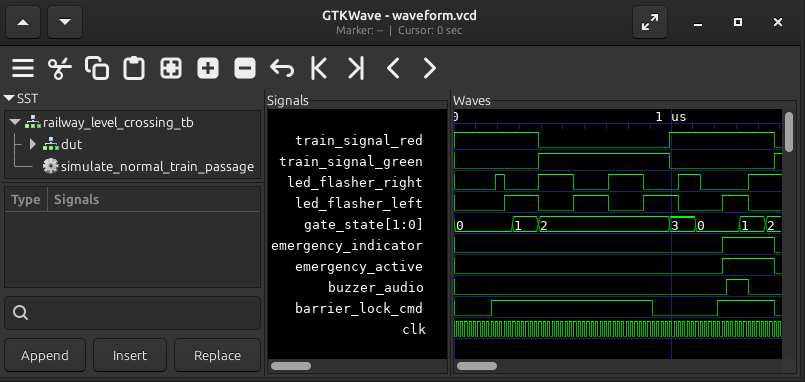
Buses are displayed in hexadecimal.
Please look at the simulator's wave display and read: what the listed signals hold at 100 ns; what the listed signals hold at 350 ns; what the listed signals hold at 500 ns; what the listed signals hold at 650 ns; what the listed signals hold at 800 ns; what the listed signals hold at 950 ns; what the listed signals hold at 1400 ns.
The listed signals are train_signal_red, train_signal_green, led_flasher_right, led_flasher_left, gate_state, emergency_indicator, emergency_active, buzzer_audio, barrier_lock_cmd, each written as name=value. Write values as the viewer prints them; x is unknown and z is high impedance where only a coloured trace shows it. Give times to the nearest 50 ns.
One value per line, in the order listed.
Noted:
train_signal_red=1, train_signal_green=0, led_flasher_right=0, led_flasher_left=0, gate_state=0, emergency_indicator=0, emergency_active=0, buzzer_audio=0, barrier_lock_cmd=0
train_signal_red=1, train_signal_green=0, led_flasher_right=0, led_flasher_left=1, gate_state=1, emergency_indicator=0, emergency_active=0, buzzer_audio=0, barrier_lock_cmd=1
train_signal_red=0, train_signal_green=1, led_flasher_right=1, led_flasher_left=0, gate_state=2, emergency_indicator=0, emergency_active=0, buzzer_audio=0, barrier_lock_cmd=1
train_signal_red=0, train_signal_green=1, led_flasher_right=0, led_flasher_left=1, gate_state=2, emergency_indicator=0, emergency_active=0, buzzer_audio=0, barrier_lock_cmd=1
train_signal_red=0, train_signal_green=1, led_flasher_right=1, led_flasher_left=0, gate_state=2, emergency_indicator=0, emergency_active=0, buzzer_audio=0, barrier_lock_cmd=1
train_signal_red=0, train_signal_green=1, led_flasher_right=0, led_flasher_left=1, gate_state=2, emergency_indicator=0, emergency_active=0, buzzer_audio=0, barrier_lock_cmd=0
train_signal_red=1, train_signal_green=0, led_flasher_right=1, led_flasher_left=0, gate_state=1, emergency_indicator=1, emergency_active=1, buzzer_audio=0, barrier_lock_cmd=1
